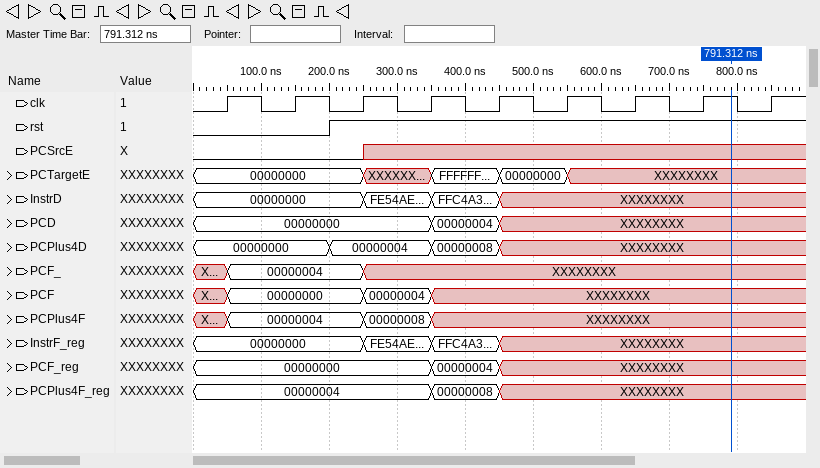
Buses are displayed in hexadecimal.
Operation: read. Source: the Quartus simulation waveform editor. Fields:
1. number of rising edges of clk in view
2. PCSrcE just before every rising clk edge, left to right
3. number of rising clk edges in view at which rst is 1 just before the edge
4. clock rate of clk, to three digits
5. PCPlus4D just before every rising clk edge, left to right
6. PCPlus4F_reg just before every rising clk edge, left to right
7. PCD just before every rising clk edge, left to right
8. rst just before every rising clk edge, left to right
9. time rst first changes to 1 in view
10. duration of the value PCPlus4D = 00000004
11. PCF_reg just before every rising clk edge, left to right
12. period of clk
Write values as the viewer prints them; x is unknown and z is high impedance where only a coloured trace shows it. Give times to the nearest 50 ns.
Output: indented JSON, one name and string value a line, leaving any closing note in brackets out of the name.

{
  "number of rising edges of clk in view": "9",
  "PCSrcE just before every rising clk edge, left to right": "0 0 0 x x x x x x",
  "number of rising clk edges in view at which rst is 1 just before the edge": "7",
  "clock rate of clk, to three digits": "10.0 MHz",
  "PCPlus4D just before every rising clk edge, left to right": "00000000, 00000000, 00000004, 00000004, 00000008, XXXXXXXX, XXXXXXXX, XXXXXXXX, XXXXXXXX",
  "PCPlus4F_reg just before every rising clk edge, left to right": "00000004, 00000004, 00000004, 00000004, 00000008, XXXXXXXX, XXXXXXXX, XXXXXXXX, XXXXXXXX",
  "PCD just before every rising clk edge, left to right": "00000000, 00000000, 00000000, 00000000, 00000004, XXXXXXXX, XXXXXXXX, XXXXXXXX, XXXXXXXX",
  "rst just before every rising clk edge, left to right": "0 0 1 1 1 1 1 1 1",
  "time rst first changes to 1 in view": "200 ns",
  "duration of the value PCPlus4D = 00000004": "150 ns",
  "PCF_reg just before every rising clk edge, left to right": "00000000, 00000000, 00000000, 00000000, 00000004, XXXXXXXX, XXXXXXXX, XXXXXXXX, XXXXXXXX",
  "period of clk": "100 ns"
}
